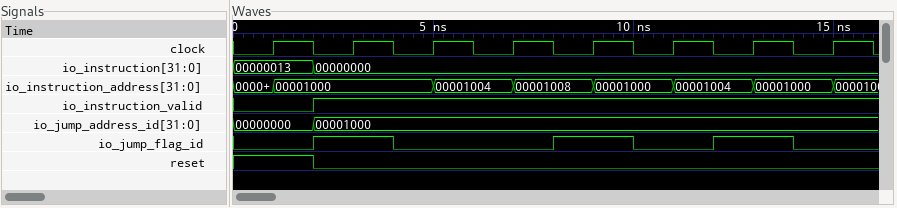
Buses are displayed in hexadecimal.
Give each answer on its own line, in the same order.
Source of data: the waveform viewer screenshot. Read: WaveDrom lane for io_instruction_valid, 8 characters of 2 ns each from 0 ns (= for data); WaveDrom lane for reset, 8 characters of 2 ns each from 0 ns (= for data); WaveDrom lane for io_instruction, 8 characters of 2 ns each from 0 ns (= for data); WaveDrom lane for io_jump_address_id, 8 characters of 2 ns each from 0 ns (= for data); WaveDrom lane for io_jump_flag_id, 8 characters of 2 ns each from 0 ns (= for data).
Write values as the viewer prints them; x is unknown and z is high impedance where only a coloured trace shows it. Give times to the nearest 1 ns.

{name: 'io_instruction_valid', wave: '01......'}
{name: 'reset', wave: '10......'}
{name: 'io_instruction', wave: '==......', data: '00000013 00000000'}
{name: 'io_jump_address_id', wave: '==......', data: '00000000 00001000'}
{name: 'io_jump_flag_id', wave: '010.1010'}
